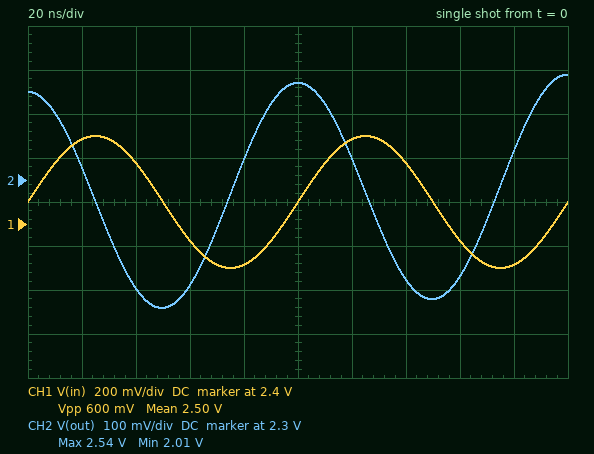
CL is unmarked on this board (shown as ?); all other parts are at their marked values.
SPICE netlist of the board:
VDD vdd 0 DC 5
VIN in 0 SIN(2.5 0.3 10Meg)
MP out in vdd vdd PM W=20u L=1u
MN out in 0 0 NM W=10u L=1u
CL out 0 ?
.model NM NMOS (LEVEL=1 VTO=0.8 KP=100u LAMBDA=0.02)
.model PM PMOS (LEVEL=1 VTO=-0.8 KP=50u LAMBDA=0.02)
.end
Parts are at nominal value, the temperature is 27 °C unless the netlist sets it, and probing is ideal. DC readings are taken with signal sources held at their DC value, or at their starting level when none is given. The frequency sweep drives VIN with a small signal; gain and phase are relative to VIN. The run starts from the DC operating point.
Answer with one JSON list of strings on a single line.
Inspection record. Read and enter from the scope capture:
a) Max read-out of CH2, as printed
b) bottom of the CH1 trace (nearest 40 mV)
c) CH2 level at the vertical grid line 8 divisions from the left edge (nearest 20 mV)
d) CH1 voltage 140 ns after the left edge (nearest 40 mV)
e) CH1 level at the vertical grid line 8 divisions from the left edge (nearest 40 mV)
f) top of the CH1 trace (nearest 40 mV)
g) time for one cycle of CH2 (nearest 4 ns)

["2.54 V", "2.20 V", "2.08 V", "2.68 V", "2.32 V", "2.80 V", "100 ns"]
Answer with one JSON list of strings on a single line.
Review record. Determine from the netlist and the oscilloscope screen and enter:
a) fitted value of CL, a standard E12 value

["68 pF"]
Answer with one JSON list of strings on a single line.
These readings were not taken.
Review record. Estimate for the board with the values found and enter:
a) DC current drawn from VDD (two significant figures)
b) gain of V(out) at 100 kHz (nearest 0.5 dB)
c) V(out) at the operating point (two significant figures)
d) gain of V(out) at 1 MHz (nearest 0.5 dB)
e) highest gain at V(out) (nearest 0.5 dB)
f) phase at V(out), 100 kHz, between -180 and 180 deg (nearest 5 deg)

["1.5 mA", "34.0 dB", "2.5 V", "18.5 dB", "36.0 dB", "145 deg"]
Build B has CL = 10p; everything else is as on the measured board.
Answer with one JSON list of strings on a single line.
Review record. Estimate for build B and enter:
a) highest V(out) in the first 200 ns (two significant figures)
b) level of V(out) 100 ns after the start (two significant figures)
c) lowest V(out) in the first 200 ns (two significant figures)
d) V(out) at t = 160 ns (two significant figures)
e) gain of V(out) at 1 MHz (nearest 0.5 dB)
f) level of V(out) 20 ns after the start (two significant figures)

["4.0 V", "3.9 V", "770 mV", "1.6 V", "32.5 dB", "1.4 V"]
